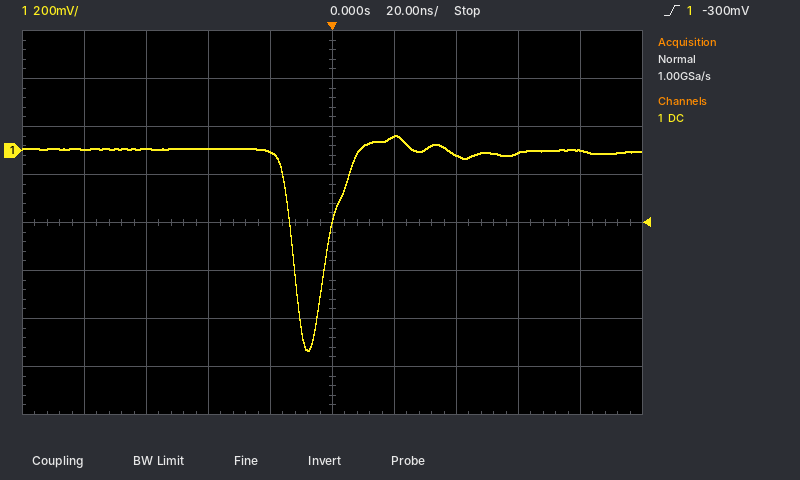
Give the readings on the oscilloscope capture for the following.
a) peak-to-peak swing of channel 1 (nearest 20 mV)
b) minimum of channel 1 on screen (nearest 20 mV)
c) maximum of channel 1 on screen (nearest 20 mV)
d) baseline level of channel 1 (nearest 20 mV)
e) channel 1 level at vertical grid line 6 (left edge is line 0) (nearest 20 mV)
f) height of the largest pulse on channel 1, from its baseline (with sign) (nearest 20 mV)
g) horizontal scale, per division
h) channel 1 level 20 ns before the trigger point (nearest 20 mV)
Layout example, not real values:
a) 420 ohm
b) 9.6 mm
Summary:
a) 900 mV
b) -840 mV
c) 60 mV
d) 0 mV
e) 60 mV
f) -840 mV
g) 20 ns
h) 0 mV
